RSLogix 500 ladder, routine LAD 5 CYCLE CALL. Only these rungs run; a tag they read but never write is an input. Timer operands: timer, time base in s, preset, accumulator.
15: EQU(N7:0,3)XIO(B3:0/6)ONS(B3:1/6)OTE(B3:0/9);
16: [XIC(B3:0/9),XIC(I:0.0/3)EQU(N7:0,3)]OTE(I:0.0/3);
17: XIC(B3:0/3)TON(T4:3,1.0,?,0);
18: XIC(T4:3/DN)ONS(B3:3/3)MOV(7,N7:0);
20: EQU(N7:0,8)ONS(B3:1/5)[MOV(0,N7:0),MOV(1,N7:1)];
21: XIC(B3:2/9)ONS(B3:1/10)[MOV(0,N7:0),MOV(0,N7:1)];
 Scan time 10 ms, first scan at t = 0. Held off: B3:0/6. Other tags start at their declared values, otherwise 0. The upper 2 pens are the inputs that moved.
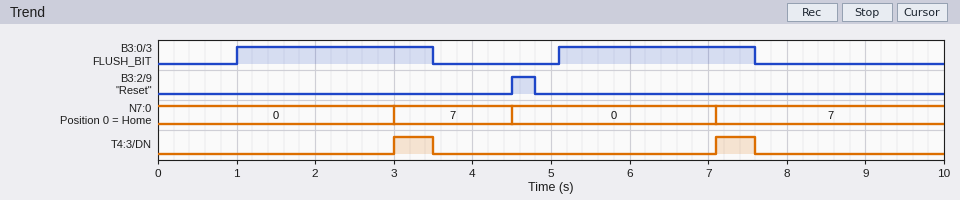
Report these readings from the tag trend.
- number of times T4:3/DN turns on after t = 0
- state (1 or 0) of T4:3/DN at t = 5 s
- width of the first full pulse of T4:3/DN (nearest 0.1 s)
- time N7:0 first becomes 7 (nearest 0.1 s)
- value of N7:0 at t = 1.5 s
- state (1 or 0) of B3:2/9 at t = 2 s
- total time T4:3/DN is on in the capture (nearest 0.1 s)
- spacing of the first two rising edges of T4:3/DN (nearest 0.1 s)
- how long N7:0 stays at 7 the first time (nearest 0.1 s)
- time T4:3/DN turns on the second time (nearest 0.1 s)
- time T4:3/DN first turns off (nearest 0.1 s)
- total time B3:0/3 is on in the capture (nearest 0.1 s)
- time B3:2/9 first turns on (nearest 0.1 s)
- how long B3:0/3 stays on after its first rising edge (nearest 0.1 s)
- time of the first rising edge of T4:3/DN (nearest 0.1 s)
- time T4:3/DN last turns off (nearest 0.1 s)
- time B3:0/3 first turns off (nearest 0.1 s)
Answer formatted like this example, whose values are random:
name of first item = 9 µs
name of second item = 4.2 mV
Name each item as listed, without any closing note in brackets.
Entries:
number of times T4:3/DN turns on after t = 0 = 2
state (1 or 0) of T4:3/DN at t = 5 s = 0
width of the first full pulse of T4:3/DN = 0.5 s
time N7:0 first becomes 7 = 3.0 s
value of N7:0 at t = 1.5 s = 0
state (1 or 0) of B3:2/9 at t = 2 s = 0
total time T4:3/DN is on in the capture = 1.0 s
spacing of the first two rising edges of T4:3/DN = 4.1 s
how long N7:0 stays at 7 the first time = 1.5 s
time T4:3/DN turns on the second time = 7.1 s
time T4:3/DN first turns off = 3.5 s
total time B3:0/3 is on in the capture = 5.0 s
time B3:2/9 first turns on = 4.5 s
how long B3:0/3 stays on after its first rising edge = 2.5 s
time of the first rising edge of T4:3/DN = 3.0 s
time T4:3/DN last turns off = 7.6 s
time B3:0/3 first turns off = 3.5 s
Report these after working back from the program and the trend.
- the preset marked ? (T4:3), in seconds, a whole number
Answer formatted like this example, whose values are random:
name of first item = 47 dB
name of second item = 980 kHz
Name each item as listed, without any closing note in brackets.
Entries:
the preset marked ? (T4:3), in seconds, a whole number = 2 s
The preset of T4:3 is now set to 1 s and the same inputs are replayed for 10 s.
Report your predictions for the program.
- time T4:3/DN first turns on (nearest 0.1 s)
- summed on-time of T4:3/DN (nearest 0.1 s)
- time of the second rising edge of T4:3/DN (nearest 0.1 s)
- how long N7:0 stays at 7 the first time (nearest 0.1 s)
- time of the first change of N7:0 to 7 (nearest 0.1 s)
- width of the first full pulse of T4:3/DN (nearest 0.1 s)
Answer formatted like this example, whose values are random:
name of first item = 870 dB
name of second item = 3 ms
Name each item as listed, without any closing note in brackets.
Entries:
time T4:3/DN first turns on = 2.0 s
summed on-time of T4:3/DN = 3.0 s
time of the second rising edge of T4:3/DN = 6.1 s
how long N7:0 stays at 7 the first time = 2.5 s
time of the first change of N7:0 to 7 = 2.0 s
width of the first full pulse of T4:3/DN = 1.5 s
